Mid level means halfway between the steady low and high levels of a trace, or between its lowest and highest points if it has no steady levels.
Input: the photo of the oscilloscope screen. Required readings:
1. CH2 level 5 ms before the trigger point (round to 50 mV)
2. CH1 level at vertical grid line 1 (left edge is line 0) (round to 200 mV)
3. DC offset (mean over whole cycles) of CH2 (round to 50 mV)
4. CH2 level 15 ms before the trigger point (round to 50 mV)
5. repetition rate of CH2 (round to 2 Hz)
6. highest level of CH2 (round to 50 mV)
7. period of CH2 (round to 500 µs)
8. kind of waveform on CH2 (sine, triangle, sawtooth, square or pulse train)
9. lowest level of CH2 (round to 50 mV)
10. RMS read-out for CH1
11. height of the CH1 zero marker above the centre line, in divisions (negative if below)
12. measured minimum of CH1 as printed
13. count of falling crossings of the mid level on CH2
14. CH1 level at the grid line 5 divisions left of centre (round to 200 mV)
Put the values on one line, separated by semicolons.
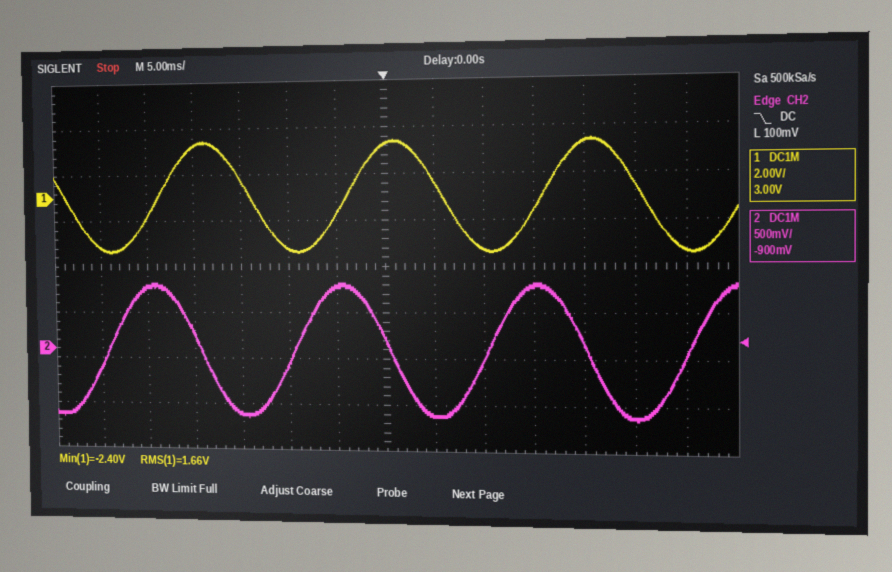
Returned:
700 mV; -2.2 V; 0 mV; -700 mV; 50 Hz; 700 mV; 20.0 ms; sine; -750 mV; 1.66 V; +1.5 div; -2.40 V; 3; -800 mV
